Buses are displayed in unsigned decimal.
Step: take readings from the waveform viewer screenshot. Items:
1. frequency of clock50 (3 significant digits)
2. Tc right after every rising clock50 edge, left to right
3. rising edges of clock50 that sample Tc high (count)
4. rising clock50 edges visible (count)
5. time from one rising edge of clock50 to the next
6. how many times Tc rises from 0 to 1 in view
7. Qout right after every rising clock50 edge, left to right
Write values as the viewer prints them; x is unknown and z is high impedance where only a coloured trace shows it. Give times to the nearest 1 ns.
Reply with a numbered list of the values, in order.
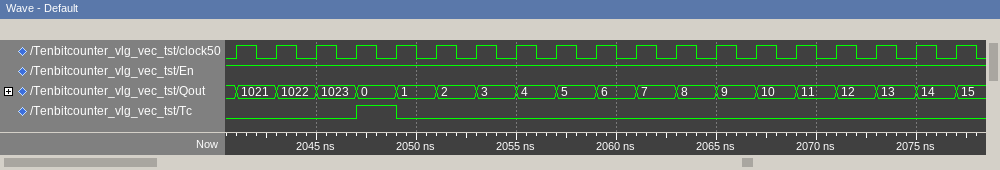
1. 500 MHz
2. 0 0 0 1 0 0 0 0 0 0 0 0 0 0 0 0 0 0 0
3. 1
4. 19
5. 2 ns
6. 1
7. 1021, 1022, 1023, 0, 1, 2, 3, 4, 5, 6, 7, 8, 9, 10, 11, 12, 13, 14, 15
